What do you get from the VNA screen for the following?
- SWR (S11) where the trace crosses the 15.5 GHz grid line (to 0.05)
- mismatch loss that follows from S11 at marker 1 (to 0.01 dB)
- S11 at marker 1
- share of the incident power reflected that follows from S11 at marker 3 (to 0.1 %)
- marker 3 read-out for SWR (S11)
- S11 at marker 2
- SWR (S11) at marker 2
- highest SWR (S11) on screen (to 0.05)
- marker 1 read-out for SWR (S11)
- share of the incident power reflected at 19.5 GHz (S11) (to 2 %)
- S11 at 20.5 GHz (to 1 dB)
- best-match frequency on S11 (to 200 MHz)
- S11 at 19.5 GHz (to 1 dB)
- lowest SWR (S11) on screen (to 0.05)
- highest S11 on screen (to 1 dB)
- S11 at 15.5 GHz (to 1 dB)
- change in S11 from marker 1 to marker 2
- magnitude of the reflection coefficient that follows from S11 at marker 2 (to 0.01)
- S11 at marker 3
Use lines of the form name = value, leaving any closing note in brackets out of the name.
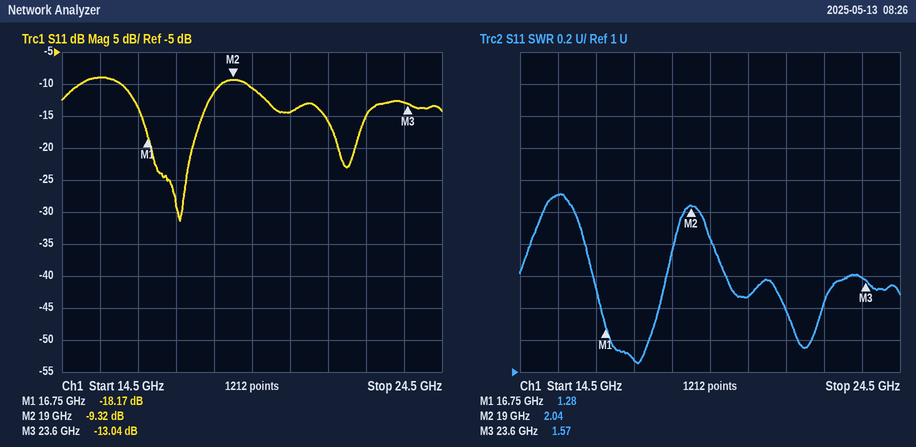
SWR (S11) where the trace crosses the 15.5 GHz grid line = 2.10
mismatch loss that follows from S11 at marker 1 = 0.07 dB
S11 at marker 1 = -18.17 dB
share of the incident power reflected that follows from S11 at marker 3 = 5.0 %
marker 3 read-out for SWR = 1.57
S11 at marker 2 = -9.32 dB
SWR (S11) at marker 2 = 2.04
highest SWR (S11) on screen = 2.10
marker 1 read-out for SWR = 1.28
share of the incident power reflected at 19.5 GHz (S11) = 8 %
S11 at 20.5 GHz = -14 dB
best-match frequency on S11 = 17.6 GHz
S11 at 19.5 GHz = -11 dB
lowest SWR (S11) on screen = 1.05
highest S11 on screen = -9 dB
S11 at 15.5 GHz = -9 dB
change in S11 from marker 1 to marker 2 = 8.85 dB
magnitude of the reflection coefficient that follows from S11 at marker 2 = 0.34
S11 at marker 3 = -13.04 dB
